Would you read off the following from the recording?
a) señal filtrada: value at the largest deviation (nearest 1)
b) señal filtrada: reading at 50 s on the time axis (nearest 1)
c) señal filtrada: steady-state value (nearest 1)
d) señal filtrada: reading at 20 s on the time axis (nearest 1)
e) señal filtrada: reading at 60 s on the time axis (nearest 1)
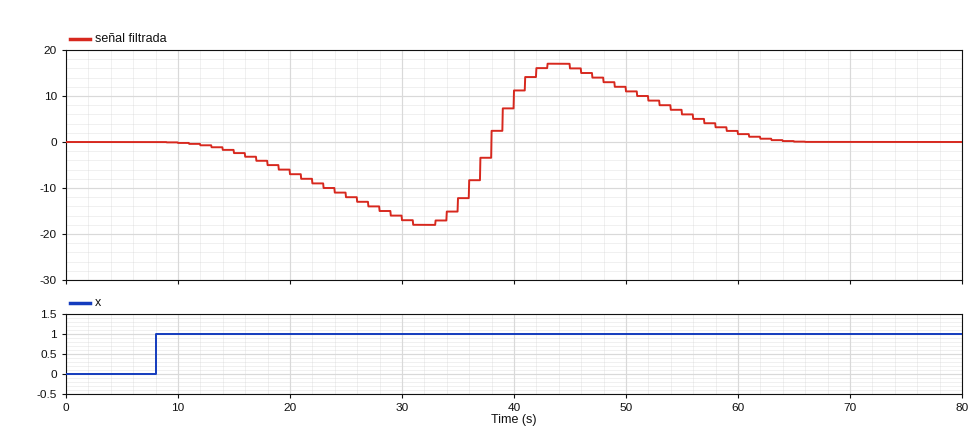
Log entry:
-18
11
0
-7
2
